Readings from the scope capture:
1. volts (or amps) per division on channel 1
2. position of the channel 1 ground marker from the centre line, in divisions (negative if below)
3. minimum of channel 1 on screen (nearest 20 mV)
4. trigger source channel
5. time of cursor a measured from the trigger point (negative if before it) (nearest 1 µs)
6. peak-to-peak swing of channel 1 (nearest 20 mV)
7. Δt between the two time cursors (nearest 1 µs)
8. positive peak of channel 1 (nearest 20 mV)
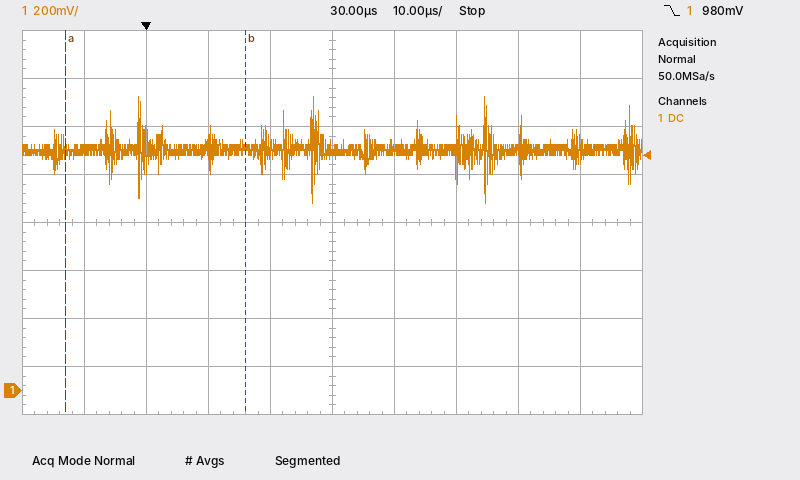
200 mV
-3.5 div
780 mV
channel 1
-13 µs
440 mV
29 µs
1.22 V
